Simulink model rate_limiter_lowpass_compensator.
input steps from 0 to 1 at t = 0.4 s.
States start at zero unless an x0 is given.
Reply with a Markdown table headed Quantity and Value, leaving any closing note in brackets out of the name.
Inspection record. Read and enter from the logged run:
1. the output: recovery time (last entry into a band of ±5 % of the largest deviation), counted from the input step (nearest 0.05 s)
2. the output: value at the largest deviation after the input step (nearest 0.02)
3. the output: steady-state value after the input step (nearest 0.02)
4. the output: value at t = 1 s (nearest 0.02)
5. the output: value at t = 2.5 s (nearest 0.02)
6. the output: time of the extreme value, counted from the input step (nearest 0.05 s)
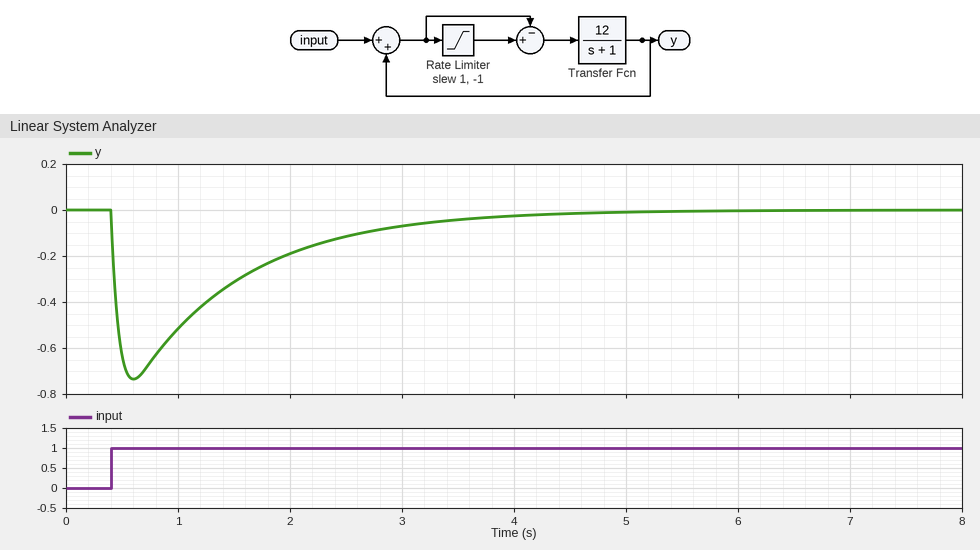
| Quantity | Value |
|---|---|
| the output: recovery time (last entry into a band of ±5 % of the largest deviation), counted from the input step | 3.25 s |
| the output: value at the largest deviation after the input step | -0.74 |
| the output: steady-state value after the input step | 0.00 |
| the output: value at t = 1 s | -0.52 |
| the output: value at t = 2.5 s | -0.12 |
| the output: time of the extreme value, counted from the input step | 0.20 s |
